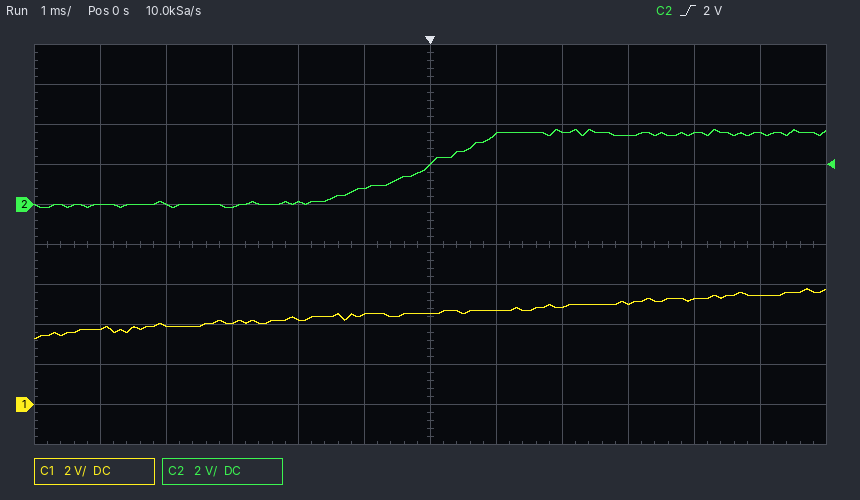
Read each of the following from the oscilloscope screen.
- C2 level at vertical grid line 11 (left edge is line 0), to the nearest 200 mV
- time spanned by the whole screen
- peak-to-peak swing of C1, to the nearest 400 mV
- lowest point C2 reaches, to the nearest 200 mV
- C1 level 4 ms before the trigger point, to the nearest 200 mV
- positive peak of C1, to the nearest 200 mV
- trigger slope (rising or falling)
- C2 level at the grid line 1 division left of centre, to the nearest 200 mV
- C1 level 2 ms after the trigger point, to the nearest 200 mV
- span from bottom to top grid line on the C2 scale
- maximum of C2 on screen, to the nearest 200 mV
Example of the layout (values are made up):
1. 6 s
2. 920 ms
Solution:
1. 3.6 V
2. 12 ms
3. 2.4 V
4. -200 mV
5. 4.0 V
6. 5.8 V
7. rising
8. 800 mV
9. 4.8 V
10. 20 V
11. 3.8 V
